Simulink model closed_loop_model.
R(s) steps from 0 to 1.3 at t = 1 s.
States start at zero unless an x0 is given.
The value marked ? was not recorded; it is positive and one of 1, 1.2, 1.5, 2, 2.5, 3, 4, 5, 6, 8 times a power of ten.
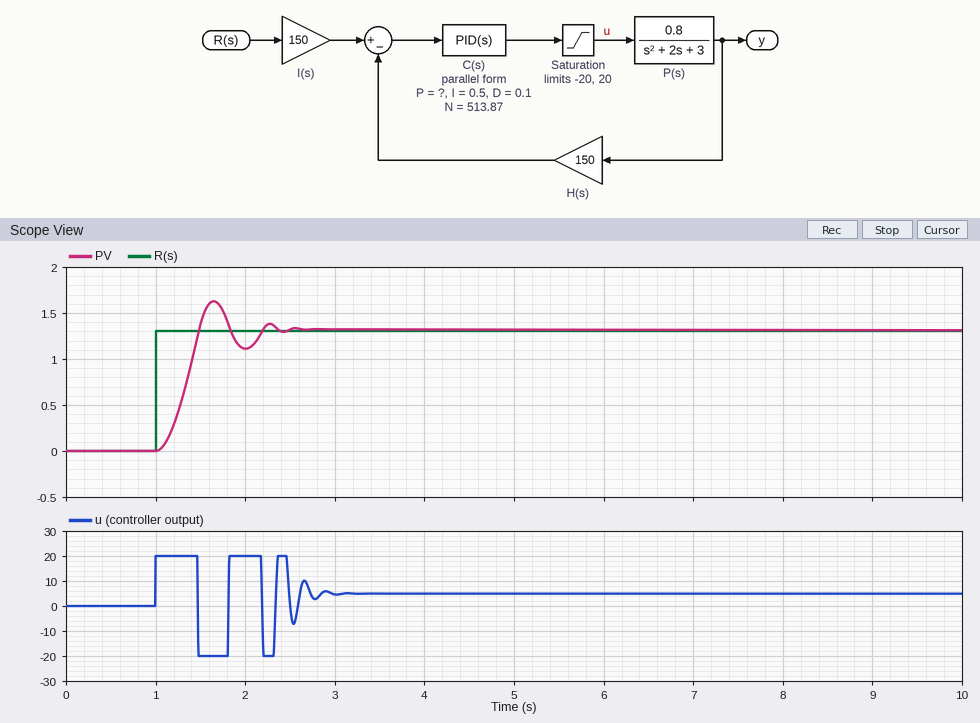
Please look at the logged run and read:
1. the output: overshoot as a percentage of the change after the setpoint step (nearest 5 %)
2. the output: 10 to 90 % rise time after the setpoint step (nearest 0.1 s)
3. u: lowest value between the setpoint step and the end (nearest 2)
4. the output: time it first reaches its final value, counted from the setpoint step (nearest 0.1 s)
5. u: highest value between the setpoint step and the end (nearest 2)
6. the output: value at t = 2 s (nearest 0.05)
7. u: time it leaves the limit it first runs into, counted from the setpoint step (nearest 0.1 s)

25 %
0.3 s
-20
0.5 s
20
1.10
0.5 s
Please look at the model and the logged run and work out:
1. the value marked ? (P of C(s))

6
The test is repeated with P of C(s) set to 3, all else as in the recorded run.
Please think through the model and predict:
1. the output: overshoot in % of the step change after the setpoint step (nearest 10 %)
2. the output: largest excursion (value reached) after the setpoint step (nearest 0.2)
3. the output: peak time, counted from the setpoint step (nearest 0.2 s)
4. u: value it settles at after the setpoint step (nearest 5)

20 %
1.6
0.6 s
5
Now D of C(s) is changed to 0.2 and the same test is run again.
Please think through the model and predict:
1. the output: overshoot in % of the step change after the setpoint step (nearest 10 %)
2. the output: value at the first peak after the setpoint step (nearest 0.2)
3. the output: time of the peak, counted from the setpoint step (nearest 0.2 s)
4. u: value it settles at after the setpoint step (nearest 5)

20 %
1.6
0.6 s
5
